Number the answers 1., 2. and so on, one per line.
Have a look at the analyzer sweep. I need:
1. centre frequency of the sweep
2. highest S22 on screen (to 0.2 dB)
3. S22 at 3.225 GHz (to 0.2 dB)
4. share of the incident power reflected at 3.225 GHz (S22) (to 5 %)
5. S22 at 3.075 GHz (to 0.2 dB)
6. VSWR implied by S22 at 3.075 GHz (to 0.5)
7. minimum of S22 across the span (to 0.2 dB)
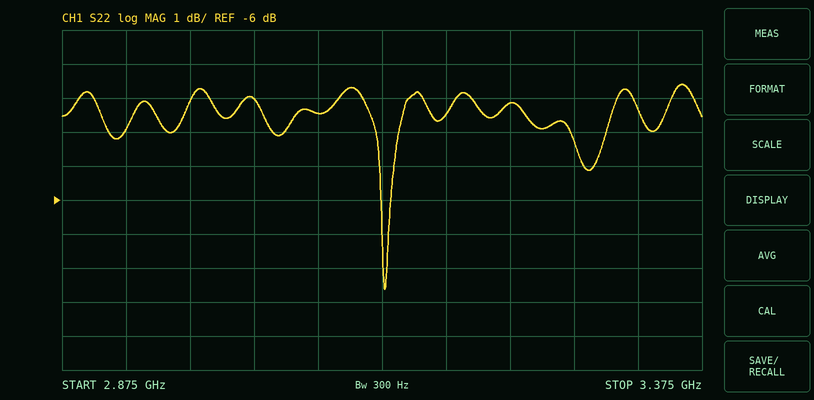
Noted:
1. 3.125 GHz
2. -2.6 dB
3. -3.2 dB
4. 50 %
5. -3.4 dB
6. 5.0
7. -8.6 dB
